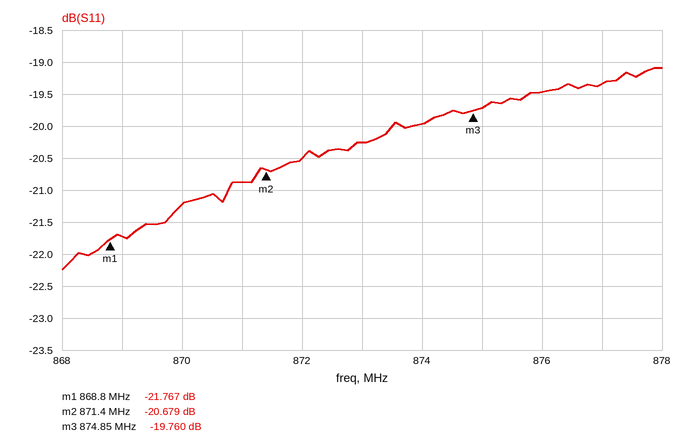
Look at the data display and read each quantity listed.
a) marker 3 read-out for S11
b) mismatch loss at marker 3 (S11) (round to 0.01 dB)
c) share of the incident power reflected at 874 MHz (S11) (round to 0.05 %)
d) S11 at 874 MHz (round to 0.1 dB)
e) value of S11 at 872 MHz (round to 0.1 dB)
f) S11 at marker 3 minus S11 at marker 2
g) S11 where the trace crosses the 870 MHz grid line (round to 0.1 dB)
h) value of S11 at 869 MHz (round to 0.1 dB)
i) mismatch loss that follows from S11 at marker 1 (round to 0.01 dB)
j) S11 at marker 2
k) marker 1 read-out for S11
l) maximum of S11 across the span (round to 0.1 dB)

-19.760 dB
0.05 dB
1.00 %
-20.0 dB
-20.5 dB
0.919 dB
-21.2 dB
-21.7 dB
0.03 dB
-20.679 dB
-21.767 dB
-19.1 dB
